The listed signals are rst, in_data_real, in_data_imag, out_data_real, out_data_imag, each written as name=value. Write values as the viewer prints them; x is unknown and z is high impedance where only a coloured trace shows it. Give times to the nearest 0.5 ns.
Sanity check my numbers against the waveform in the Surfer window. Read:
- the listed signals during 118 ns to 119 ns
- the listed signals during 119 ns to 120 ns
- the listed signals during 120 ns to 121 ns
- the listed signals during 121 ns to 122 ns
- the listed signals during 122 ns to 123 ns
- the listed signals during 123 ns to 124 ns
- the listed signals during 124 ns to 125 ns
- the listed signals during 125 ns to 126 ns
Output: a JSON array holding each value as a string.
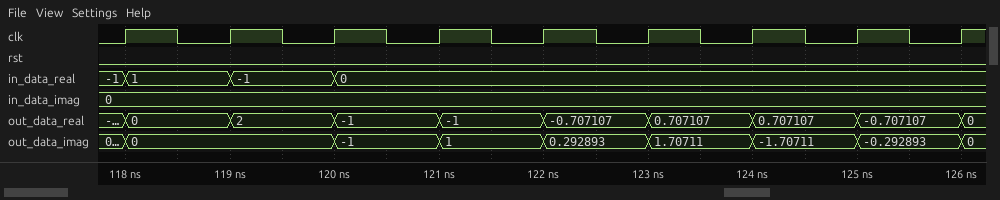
["rst=0, in_data_real=1, in_data_imag=0, out_data_real=0, out_data_imag=0", "rst=0, in_data_real=-1, in_data_imag=0, out_data_real=2, out_data_imag=0", "rst=0, in_data_real=0, in_data_imag=0, out_data_real=-1, out_data_imag=-1", "rst=0, in_data_real=0, in_data_imag=0, out_data_real=-1, out_data_imag=1", "rst=0, in_data_real=0, in_data_imag=0, out_data_real=-0.707107, out_data_imag=0.292893", "rst=0, in_data_real=0, in_data_imag=0, out_data_real=0.707107, out_data_imag=1.70711", "rst=0, in_data_real=0, in_data_imag=0, out_data_real=0.707107, out_data_imag=-1.70711", "rst=0, in_data_real=0, in_data_imag=0, out_data_real=-0.707107, out_data_imag=-0.292893"]
